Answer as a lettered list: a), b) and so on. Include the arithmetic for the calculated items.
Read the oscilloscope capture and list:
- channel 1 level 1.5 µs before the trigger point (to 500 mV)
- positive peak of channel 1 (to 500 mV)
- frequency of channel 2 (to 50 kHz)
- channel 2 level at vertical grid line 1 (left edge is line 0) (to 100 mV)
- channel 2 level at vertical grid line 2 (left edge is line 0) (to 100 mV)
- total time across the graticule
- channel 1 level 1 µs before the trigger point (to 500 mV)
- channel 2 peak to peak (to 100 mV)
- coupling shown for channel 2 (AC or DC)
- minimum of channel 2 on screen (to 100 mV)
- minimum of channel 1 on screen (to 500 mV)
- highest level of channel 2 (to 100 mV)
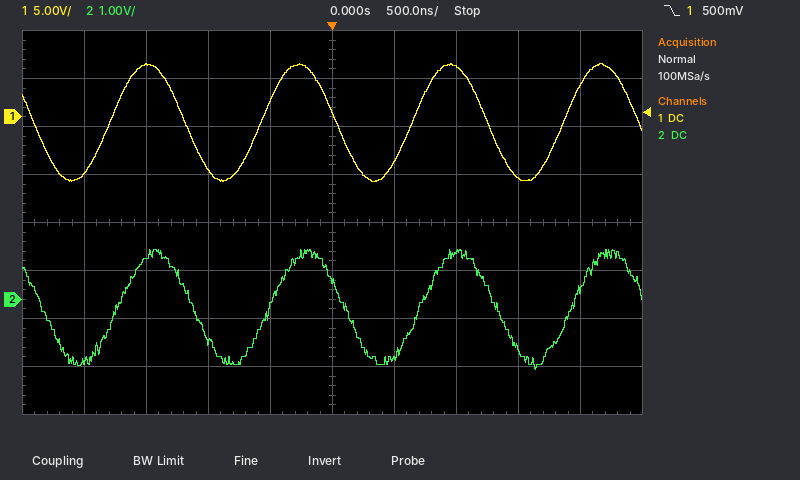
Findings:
a) 5.5 V
b) 5.5 V
c) 800 kHz
d) -1.3 V
e) 900 mV
f) 5 µs
g) -5.5 V
h) 1.0 V − (-1.5 V) = 2.5 V
i) DC
j) -1.5 V
k) -6.5 V
l) 1.0 V
